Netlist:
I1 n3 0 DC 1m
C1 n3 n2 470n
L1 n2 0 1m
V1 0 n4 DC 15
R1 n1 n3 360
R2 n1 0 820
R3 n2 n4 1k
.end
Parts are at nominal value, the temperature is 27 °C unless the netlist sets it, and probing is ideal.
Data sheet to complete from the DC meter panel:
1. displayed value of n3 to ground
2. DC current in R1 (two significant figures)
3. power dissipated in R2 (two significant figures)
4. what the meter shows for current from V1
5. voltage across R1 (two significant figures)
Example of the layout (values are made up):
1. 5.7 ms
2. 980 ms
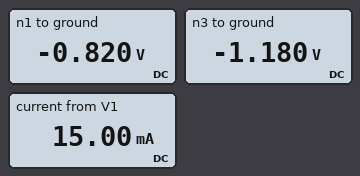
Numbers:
1. -1.180 V
2. 1.0 mA
3. 820 µW
4. 15.00 mA
5. 360 mV
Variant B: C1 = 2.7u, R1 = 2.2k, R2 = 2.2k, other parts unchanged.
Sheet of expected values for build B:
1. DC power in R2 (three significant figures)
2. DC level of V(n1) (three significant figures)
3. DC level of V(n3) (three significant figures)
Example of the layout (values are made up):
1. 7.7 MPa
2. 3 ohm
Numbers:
1. 2.20 mW
2. -2.20 V
3. -4.40 V
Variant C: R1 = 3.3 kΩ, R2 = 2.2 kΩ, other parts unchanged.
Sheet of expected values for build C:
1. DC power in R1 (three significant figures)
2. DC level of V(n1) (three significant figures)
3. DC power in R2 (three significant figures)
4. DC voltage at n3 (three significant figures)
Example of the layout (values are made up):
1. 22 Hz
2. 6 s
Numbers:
1. 3.30 mW
2. -2.20 V
3. 2.20 mW
4. -5.50 V
